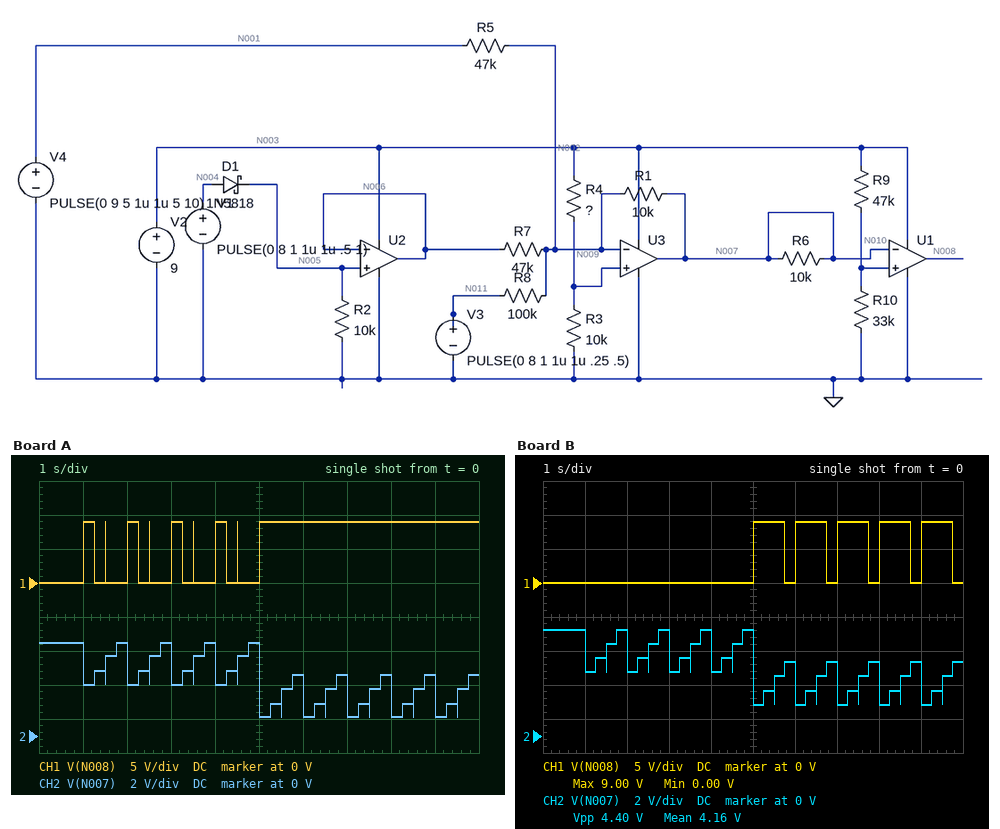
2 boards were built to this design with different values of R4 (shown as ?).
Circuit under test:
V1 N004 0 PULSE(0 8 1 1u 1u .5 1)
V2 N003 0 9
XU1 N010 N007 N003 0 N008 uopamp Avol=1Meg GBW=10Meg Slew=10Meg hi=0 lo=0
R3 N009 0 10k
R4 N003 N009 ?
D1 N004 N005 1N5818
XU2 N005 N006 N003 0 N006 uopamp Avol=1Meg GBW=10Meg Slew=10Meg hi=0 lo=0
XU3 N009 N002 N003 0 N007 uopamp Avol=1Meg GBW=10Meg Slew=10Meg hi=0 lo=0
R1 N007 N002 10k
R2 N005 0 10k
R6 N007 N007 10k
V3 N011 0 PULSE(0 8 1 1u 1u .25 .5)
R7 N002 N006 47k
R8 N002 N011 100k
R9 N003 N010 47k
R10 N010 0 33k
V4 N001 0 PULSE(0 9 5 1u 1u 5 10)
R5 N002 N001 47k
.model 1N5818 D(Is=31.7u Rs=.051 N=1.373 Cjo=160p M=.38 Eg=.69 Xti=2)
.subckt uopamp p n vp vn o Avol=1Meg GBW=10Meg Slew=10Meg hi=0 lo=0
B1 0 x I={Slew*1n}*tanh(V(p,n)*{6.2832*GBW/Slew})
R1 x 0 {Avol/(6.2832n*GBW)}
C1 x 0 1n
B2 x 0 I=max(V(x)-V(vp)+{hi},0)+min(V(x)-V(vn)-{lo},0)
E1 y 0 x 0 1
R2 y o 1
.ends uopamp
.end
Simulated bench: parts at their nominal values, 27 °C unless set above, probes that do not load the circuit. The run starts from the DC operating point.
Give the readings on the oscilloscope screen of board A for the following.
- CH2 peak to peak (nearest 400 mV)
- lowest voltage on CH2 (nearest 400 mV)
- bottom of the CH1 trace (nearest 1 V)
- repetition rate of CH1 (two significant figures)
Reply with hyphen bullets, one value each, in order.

- 4.4 V
- 1.2 V
- 0 V
- 1.0 Hz
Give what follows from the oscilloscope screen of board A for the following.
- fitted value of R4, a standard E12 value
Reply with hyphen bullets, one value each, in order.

- 15 kΩ
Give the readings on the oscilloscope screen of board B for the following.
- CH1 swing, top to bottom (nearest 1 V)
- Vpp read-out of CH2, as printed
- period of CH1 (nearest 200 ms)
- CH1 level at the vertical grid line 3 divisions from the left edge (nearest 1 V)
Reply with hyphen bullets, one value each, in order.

- 9 V
- 4.40 V
- 1.0 s
- 0 V
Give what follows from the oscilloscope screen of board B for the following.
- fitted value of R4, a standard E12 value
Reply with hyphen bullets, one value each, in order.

- 12 kΩ
